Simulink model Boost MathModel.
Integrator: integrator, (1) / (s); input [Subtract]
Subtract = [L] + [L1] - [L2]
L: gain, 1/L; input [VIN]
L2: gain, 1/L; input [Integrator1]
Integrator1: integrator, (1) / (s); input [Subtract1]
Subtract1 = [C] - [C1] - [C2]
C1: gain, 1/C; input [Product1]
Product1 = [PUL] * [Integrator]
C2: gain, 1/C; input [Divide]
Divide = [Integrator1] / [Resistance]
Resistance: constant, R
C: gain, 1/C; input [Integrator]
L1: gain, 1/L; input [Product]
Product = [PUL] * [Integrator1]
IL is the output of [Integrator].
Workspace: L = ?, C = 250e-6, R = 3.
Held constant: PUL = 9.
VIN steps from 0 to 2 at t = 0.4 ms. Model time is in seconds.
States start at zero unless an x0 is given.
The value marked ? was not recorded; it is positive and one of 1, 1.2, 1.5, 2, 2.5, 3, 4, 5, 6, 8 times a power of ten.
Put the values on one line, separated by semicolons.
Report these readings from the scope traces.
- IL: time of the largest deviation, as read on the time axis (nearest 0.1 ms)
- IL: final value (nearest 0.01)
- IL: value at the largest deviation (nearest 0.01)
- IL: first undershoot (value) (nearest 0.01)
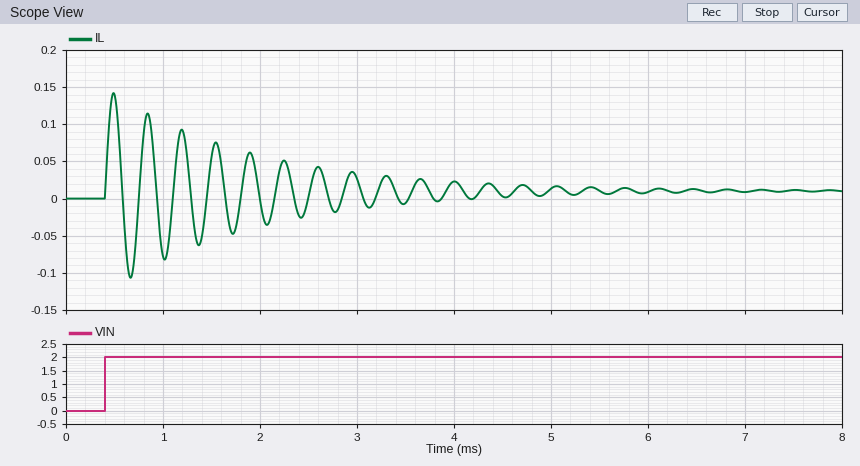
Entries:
0.5 ms; 0.01; 0.14; -0.11
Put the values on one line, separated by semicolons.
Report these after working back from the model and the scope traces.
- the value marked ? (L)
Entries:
0.0008
